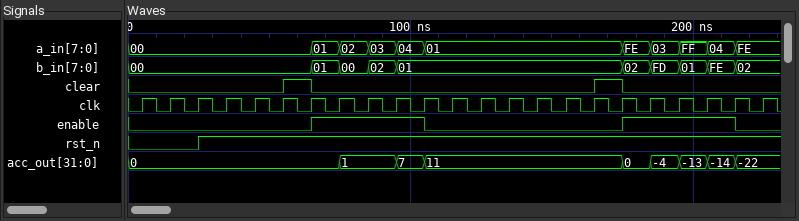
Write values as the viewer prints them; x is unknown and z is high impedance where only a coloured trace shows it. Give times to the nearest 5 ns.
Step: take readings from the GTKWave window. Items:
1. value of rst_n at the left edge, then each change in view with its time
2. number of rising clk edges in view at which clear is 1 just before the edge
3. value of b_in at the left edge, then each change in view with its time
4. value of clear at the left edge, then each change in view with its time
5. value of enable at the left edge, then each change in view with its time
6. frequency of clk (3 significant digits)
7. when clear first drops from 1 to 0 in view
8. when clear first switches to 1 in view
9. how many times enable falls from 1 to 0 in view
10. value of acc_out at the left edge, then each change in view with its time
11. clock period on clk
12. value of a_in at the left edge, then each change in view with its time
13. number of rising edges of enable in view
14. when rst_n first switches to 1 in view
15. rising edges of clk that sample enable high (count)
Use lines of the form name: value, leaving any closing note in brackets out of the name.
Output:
value of rst_n at the left edge, then each change in view with its time: 0, 1 at 25 ns
number of rising clk edges in view at which clear is 1 just before the edge: 2
value of b_in at the left edge, then each change in view with its time: 00, 01 at 65 ns, 00 at 75 ns, 02 at 85 ns, 01 at 95 ns, 02 at 175 ns, FD at 185 ns, 01 at 195 ns, FE at 205 ns, 02 at 215 ns
value of clear at the left edge, then each change in view with its time: 0, 1 at 55 ns, 0 at 65 ns, 1 at 165 ns, 0 at 175 ns
value of enable at the left edge, then each change in view with its time: 0, 1 at 65 ns, 0 at 105 ns, 1 at 175 ns, 0 at 215 ns
frequency of clk: 100 MHz
when clear first drops from 1 to 0 in view: 65 ns
when clear first switches to 1 in view: 55 ns
how many times enable falls from 1 to 0 in view: 2
value of acc_out at the left edge, then each change in view with its time: 0, 1 at 75 ns, 7 at 95 ns, 11 at 105 ns, 0 at 175 ns, -4 at 185 ns, -13 at 195 ns, -14 at 205 ns, -22 at 215 ns
clock period on clk: 10 ns
value of a_in at the left edge, then each change in view with its time: 00, 01 at 65 ns, 02 at 75 ns, 03 at 85 ns, 04 at 95 ns, 01 at 105 ns, FE at 175 ns, 03 at 185 ns, FF at 195 ns, 04 at 205 ns, FE at 215 ns
number of rising edges of enable in view: 2
when rst_n first switches to 1 in view: 25 ns
rising edges of clk that sample enable high: 8
